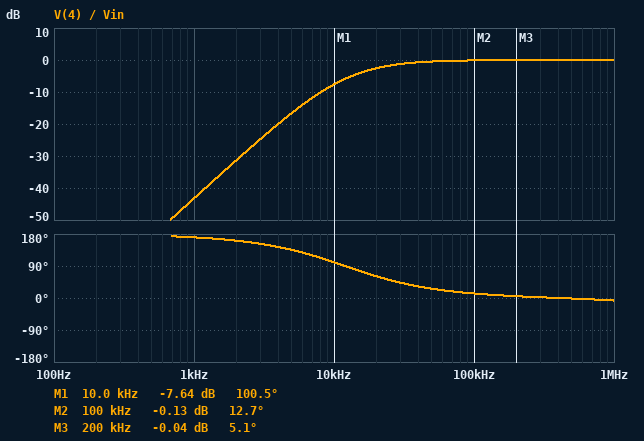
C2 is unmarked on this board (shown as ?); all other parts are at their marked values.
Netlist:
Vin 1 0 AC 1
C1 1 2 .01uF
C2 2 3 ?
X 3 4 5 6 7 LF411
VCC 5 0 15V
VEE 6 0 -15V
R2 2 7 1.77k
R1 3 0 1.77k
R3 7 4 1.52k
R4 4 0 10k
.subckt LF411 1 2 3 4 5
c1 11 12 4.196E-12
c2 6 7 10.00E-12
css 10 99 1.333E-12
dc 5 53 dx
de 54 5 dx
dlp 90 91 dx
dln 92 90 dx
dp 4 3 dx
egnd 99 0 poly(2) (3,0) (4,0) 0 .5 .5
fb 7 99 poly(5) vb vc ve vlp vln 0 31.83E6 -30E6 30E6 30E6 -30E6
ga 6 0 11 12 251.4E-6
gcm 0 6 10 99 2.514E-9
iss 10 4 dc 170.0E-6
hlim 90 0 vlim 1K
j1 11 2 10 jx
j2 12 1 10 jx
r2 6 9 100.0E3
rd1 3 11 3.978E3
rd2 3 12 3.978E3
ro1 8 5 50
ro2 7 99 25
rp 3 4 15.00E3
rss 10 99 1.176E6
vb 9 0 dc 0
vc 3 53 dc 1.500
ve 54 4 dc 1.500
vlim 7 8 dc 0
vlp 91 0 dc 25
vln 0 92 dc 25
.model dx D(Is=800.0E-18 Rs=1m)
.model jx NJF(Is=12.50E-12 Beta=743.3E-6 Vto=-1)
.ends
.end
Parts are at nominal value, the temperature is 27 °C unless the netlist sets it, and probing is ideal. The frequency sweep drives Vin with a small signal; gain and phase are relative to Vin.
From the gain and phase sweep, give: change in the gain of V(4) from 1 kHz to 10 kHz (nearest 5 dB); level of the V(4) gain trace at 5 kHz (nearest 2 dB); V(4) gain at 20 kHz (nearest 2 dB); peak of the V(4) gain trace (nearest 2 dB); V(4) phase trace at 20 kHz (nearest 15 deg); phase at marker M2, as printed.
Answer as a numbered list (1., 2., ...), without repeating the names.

1. 35 dB
2. -16 dB
3. -2 dB
4. 0 dB
5. 60 deg
6. 12.7 deg
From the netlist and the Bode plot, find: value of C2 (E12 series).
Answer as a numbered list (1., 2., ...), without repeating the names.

1. 5.6 nF
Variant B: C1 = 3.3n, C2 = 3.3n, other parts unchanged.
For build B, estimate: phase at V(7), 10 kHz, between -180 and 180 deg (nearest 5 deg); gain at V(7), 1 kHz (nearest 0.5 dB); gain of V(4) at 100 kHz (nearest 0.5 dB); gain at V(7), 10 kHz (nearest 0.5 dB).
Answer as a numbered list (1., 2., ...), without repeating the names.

1. 140 deg
2. -56.0 dB
3. -0.5 dB
4. -17.0 dB
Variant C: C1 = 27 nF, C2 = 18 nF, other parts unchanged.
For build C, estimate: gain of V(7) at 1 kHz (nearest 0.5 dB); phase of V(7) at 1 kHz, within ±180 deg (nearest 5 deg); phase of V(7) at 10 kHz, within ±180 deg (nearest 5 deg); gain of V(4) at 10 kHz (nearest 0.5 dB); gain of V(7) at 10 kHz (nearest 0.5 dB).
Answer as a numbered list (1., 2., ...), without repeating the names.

1. -23.5 dB
2. 155 deg
3. 45 deg
4. -1.0 dB
5. 0 dB
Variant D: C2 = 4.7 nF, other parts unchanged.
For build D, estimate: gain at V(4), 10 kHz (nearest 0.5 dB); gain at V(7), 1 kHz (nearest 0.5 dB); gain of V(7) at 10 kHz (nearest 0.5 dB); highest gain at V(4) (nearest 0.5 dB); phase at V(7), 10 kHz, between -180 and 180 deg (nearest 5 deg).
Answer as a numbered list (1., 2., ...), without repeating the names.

1. -9.0 dB
2. -43.5 dB
3. -7.5 dB
4. 2.0 dB
5. 105 deg
